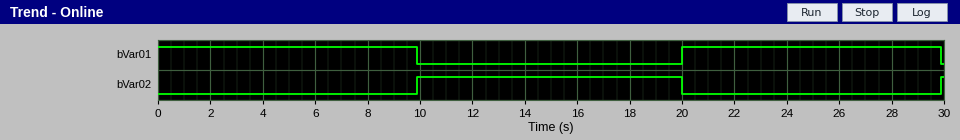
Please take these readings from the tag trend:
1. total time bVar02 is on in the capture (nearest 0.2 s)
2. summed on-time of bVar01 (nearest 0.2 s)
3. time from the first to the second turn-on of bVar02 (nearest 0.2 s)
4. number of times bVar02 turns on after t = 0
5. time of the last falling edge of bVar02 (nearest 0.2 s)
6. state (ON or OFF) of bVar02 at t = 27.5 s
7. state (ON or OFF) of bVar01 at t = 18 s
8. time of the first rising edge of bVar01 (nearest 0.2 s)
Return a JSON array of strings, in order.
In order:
["10.2 s", "19.8 s", "20.0 s", "2", "20.0 s", "OFF", "OFF", "20.0 s"]
